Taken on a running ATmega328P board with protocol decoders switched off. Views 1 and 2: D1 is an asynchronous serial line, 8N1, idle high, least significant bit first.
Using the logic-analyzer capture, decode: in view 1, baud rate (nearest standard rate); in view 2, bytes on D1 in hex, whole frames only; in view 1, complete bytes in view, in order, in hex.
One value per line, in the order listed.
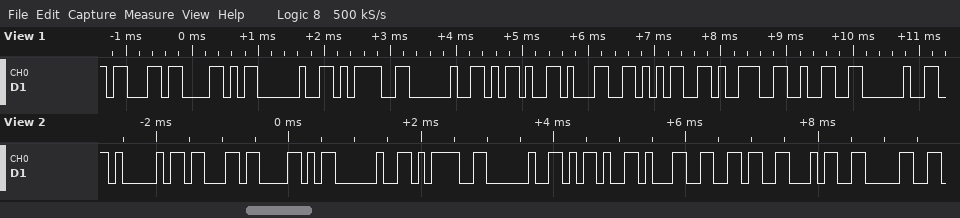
9600 baud
0x41 0x63 0x58 0x20 0x3D 0x20 0x2D 0x31 0x36 0x34 0x30
63 58 20 3D 20 2D 31 35 39 32 20
